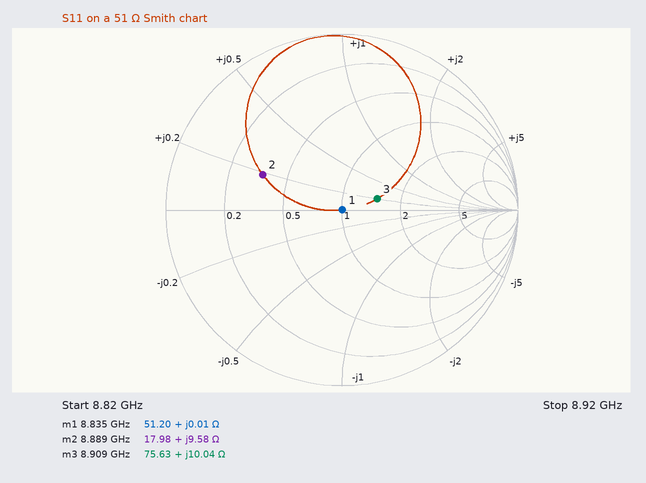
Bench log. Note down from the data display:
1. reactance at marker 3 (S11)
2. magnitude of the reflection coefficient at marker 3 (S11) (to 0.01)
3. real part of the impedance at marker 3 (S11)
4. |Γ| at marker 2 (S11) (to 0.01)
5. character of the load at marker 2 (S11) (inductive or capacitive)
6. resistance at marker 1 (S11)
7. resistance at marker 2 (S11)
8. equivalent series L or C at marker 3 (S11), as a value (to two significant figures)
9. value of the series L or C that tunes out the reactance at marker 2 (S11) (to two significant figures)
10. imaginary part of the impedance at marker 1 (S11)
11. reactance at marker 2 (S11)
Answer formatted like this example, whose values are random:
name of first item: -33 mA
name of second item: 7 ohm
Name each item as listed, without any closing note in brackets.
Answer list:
reactance at marker 3: +10.04 Ω
magnitude of the reflection coefficient at marker 3 (S11): 0.21
real part of the impedance at marker 3: 75.63 Ω
|Γ| at marker 2 (S11): 0.49
character of the load at marker 2 (S11): inductive
resistance at marker 1: 51.20 Ω
resistance at marker 2: 17.98 Ω
equivalent series L or C at marker 3 (S11), as a value: 180 pH
value of the series L or C that tunes out the reactance at marker 2 (S11): 1.9 pF
imaginary part of the impedance at marker 1: +0.01 Ω
reactance at marker 2: +9.58 Ω
